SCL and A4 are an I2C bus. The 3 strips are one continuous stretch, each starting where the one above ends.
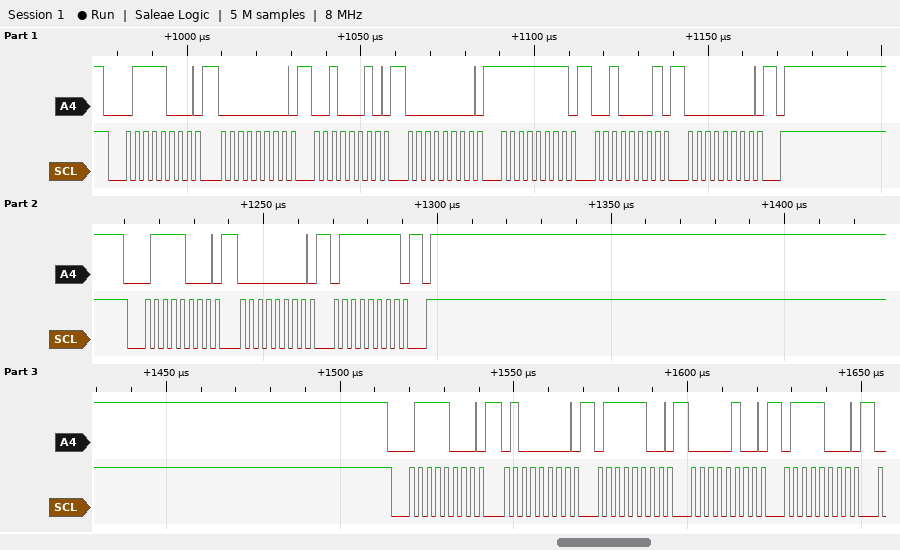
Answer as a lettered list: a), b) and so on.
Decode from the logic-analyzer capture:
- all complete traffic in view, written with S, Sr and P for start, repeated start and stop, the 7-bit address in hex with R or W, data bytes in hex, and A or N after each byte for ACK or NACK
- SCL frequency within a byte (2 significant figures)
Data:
a) S 3CW A 00 A 22 A 00 A FF A 21 A 00 A P S 3CW A 00 A 7F A P S 3CW A 40 A 7C A 04 A 78 A
b) 400 kHz
